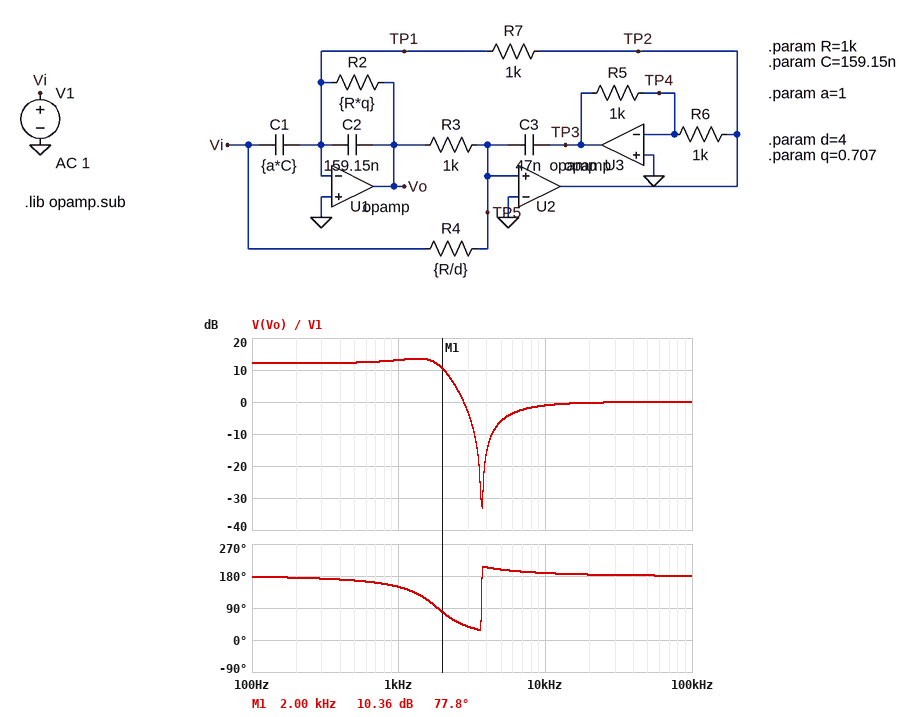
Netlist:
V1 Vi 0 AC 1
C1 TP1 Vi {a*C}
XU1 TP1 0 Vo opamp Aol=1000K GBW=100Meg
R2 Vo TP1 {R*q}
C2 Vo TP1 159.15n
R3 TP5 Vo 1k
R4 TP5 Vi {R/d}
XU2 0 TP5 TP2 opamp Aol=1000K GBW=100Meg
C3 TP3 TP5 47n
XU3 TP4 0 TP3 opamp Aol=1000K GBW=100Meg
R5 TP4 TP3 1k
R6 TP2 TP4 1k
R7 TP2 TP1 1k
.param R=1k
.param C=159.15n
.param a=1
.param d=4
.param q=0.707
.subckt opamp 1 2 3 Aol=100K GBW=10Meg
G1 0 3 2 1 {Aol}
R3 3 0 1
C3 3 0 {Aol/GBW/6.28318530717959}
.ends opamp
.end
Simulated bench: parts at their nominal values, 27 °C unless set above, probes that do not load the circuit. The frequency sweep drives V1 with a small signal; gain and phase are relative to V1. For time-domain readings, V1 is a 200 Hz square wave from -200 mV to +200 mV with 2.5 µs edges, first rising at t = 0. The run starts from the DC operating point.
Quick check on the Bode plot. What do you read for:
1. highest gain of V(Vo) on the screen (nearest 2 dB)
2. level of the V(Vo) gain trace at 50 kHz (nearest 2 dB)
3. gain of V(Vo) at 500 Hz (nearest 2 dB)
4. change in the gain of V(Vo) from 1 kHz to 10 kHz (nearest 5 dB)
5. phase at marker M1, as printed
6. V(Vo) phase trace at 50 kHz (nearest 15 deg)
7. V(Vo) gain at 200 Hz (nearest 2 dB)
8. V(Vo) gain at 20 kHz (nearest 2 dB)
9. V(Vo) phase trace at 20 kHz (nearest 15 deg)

14 dB
0 dB
12 dB
-15 dB
77.8 deg
180 deg
12 dB
0 dB
180 deg
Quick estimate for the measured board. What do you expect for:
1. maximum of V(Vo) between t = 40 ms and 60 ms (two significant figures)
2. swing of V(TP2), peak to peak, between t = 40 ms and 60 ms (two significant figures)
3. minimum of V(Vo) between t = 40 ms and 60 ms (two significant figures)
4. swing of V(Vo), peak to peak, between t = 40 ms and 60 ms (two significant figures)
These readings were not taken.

1.1 V
4.3 V
-1.1 V
2.3 V
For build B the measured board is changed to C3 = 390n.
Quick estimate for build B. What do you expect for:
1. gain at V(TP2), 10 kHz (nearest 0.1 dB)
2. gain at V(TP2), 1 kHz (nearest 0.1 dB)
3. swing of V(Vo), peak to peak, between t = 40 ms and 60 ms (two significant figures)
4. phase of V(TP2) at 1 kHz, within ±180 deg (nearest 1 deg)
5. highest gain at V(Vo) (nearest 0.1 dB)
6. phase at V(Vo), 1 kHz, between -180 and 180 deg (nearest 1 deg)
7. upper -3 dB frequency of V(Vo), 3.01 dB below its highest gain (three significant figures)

-18.1 dB
4.6 dB
1.6 V
-85 deg
12.0 dB
67 deg
315 Hz
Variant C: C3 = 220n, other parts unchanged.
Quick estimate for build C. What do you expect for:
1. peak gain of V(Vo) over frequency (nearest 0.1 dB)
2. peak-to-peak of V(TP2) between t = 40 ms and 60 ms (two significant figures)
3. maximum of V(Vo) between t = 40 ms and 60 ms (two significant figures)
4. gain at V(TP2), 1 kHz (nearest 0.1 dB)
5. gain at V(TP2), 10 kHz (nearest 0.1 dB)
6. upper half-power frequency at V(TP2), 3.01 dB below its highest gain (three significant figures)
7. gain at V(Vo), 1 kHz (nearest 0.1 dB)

12.0 dB
2.3 V
810 mV
10.1 dB
-13.1 dB
778 Hz
2.4 dB
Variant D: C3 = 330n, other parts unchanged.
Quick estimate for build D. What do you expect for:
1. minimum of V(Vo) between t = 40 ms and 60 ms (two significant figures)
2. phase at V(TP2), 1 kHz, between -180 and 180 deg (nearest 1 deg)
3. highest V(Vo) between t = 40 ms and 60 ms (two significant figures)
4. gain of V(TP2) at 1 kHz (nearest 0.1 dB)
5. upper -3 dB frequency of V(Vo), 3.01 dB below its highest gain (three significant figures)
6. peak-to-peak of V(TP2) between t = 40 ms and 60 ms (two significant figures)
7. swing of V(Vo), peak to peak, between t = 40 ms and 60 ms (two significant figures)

-800 mV
-82 deg
800 mV
6.2 dB
376 Hz
2.3 V
1.6 V
